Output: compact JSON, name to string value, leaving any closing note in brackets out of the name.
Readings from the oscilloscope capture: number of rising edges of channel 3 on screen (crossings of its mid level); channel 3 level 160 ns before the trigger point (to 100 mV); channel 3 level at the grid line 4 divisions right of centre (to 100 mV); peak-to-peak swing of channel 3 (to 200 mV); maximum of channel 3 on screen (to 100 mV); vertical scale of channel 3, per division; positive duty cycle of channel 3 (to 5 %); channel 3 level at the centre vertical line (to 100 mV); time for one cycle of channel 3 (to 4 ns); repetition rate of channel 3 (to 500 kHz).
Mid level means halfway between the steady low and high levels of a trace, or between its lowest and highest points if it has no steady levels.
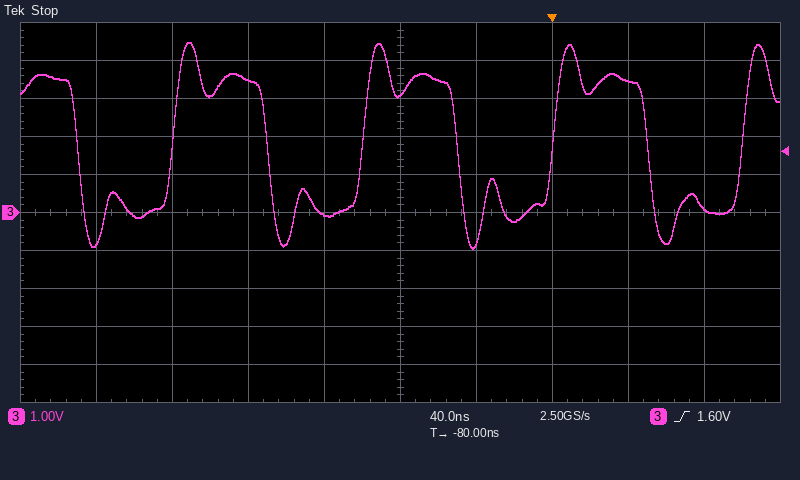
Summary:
{"number of rising edges of channel 3 on screen": "4", "channel 3 level 160 ns before the trigger point": "3.5 V", "channel 3 level at the grid line 4 divisions right of centre": "100 mV", "peak-to-peak swing of channel 3": "5.4 V", "maximum of channel 3 on screen": "4.5 V", "vertical scale of channel 3, per division": "1 V", "positive duty cycle of channel 3": "50 %", "channel 3 level at the centre vertical line": "3.1 V", "time for one cycle of channel 3": "100 ns", "repetition rate of channel 3": "10.0 MHz"}
